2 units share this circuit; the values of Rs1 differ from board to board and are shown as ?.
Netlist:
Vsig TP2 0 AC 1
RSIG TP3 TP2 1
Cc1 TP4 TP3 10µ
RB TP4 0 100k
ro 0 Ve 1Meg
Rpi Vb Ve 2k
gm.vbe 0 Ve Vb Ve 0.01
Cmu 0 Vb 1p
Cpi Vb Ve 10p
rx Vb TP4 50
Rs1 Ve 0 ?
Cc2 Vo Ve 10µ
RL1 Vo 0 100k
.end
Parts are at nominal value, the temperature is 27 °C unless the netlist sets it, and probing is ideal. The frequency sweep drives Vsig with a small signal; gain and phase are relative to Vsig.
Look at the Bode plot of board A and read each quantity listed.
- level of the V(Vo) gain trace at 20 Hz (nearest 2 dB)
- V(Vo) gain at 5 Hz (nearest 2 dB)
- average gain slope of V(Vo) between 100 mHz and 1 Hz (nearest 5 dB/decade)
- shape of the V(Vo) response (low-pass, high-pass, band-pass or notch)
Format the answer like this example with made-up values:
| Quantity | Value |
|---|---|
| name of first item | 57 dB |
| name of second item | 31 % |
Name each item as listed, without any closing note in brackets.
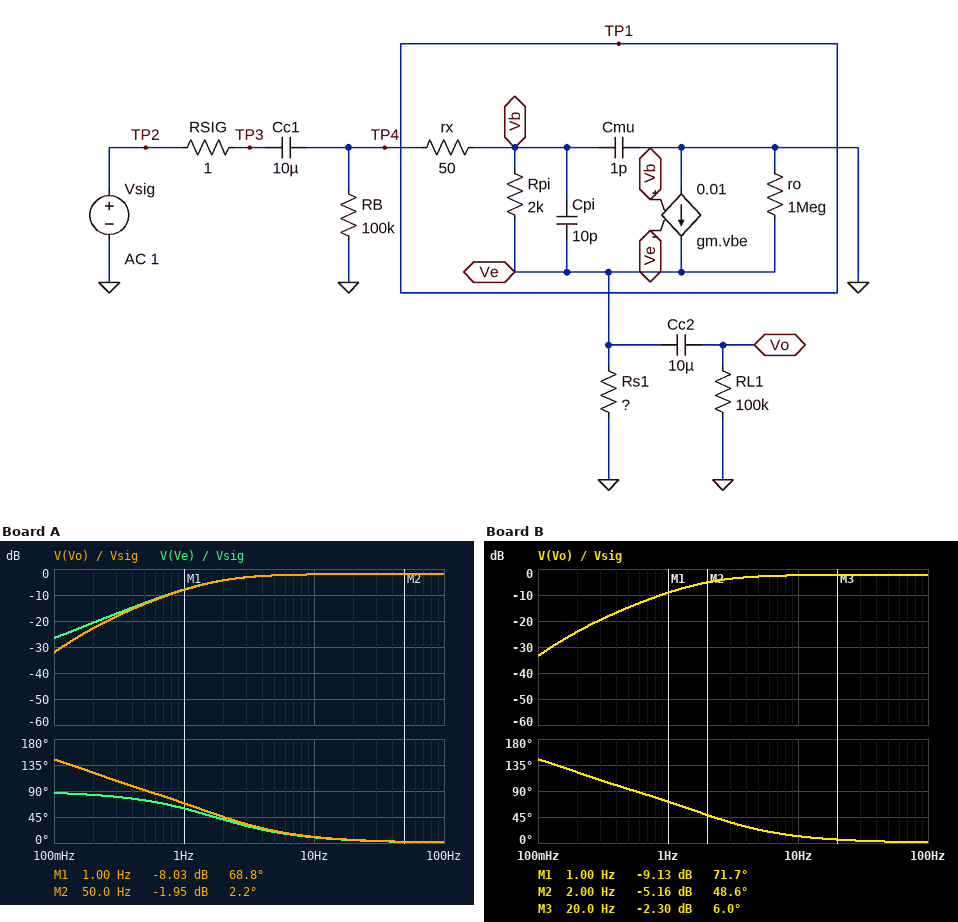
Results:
| Quantity | Value |
|---|---|
| level of the V(Vo) gain trace at 20 Hz | -2 dB |
| V(Vo) gain at 5 Hz | -2 dB |
| average gain slope of V(Vo) between 100 mHz and 1 Hz | 25 dB/decade |
| shape of the V(Vo) response | high-pass |
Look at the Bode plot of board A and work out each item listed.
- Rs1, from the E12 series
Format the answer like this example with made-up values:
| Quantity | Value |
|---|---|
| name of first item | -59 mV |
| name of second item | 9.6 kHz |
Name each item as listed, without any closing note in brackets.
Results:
| Quantity | Value |
|---|---|
| Rs1, from the E12 series | 390 Ω |
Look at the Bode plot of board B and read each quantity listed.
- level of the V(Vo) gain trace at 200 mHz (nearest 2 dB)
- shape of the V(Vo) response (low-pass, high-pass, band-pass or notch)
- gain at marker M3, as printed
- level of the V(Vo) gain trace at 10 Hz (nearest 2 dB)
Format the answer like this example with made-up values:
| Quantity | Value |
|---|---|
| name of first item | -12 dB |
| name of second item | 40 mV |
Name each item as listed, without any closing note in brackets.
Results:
| Quantity | Value |
|---|---|
| level of the V(Vo) gain trace at 200 mHz | -24 dB |
| shape of the V(Vo) response | high-pass |
| gain at marker M3, as printed | -2.30 dB |
| level of the V(Vo) gain trace at 10 Hz | -2 dB |
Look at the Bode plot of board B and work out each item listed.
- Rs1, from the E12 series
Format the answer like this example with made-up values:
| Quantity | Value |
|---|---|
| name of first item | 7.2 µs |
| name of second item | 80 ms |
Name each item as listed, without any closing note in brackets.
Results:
| Quantity | Value |
|---|---|
| Rs1, from the E12 series | 330 Ω |
